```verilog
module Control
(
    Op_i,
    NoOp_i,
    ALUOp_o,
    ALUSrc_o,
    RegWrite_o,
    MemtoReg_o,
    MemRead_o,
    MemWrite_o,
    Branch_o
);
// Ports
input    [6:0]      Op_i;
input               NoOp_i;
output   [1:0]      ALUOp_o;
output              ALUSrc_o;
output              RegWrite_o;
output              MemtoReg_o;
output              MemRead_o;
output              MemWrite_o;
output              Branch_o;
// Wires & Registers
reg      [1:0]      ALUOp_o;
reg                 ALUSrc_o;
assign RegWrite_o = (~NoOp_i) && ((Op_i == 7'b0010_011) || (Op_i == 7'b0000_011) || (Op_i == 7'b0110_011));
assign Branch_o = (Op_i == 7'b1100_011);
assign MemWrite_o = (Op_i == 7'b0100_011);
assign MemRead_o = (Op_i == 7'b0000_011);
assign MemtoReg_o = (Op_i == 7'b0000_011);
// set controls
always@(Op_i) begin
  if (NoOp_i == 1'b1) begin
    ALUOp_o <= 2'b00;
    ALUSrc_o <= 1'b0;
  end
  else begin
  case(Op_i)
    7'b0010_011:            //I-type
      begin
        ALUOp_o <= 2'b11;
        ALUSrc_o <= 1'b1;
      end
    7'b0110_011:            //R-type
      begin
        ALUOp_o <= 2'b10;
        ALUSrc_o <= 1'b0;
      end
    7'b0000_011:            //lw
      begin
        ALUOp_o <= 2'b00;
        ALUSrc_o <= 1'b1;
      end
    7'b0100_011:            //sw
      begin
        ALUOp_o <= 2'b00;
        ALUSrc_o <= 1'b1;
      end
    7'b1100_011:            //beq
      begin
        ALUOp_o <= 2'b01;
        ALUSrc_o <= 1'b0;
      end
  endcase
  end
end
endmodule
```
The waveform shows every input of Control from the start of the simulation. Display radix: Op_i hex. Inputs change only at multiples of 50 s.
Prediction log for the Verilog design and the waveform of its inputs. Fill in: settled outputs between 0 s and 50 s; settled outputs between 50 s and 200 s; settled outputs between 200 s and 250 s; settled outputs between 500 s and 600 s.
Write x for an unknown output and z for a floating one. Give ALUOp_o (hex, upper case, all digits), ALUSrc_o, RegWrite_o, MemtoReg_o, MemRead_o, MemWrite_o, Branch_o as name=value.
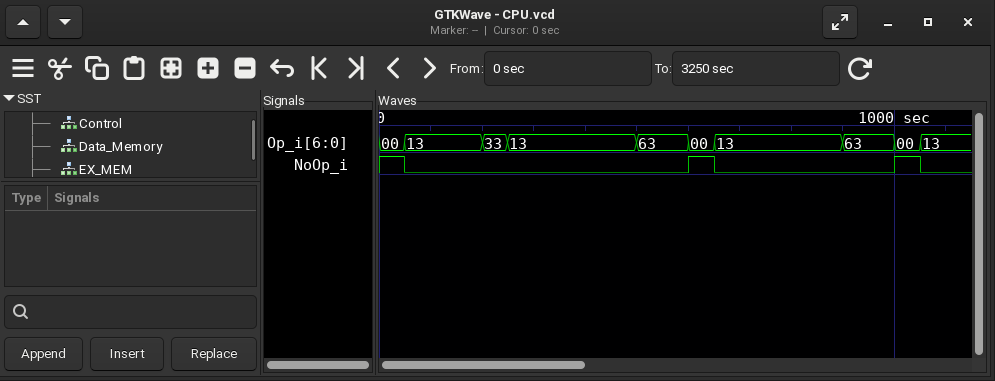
ALUOp_o=0, ALUSrc_o=0, RegWrite_o=0, MemtoReg_o=0, MemRead_o=0, MemWrite_o=0, Branch_o=0
ALUOp_o=3, ALUSrc_o=1, RegWrite_o=1, MemtoReg_o=0, MemRead_o=0, MemWrite_o=0, Branch_o=0
ALUOp_o=2, ALUSrc_o=0, RegWrite_o=1, MemtoReg_o=0, MemRead_o=0, MemWrite_o=0, Branch_o=0
ALUOp_o=1, ALUSrc_o=0, RegWrite_o=0, MemtoReg_o=0, MemRead_o=0, MemWrite_o=0, Branch_o=1
